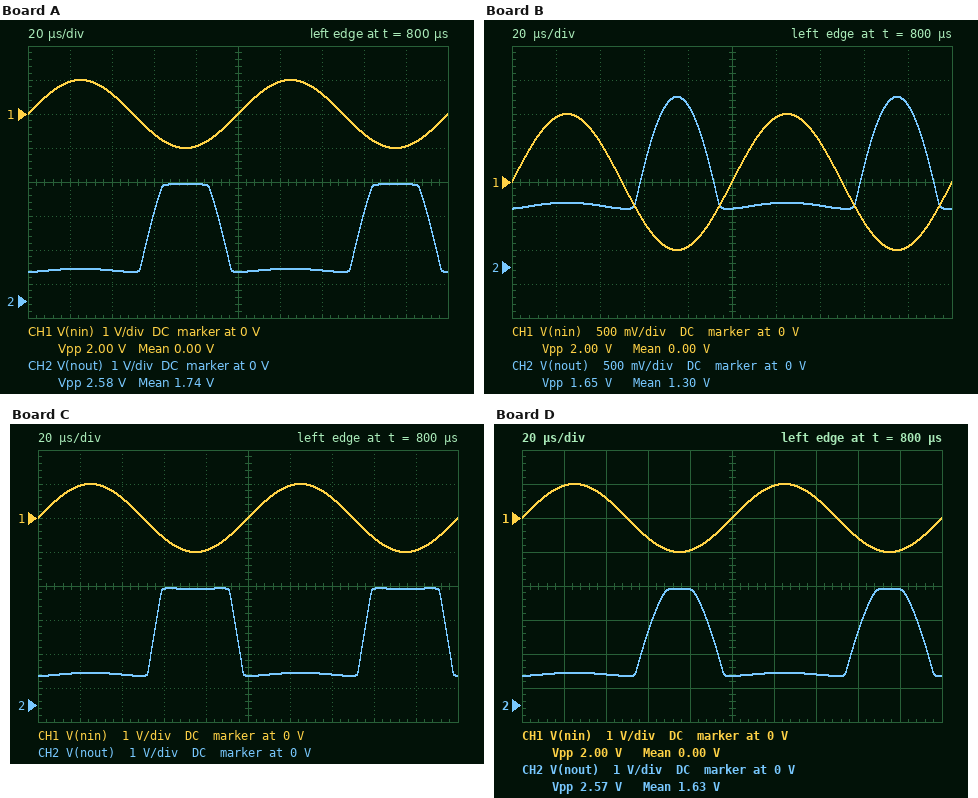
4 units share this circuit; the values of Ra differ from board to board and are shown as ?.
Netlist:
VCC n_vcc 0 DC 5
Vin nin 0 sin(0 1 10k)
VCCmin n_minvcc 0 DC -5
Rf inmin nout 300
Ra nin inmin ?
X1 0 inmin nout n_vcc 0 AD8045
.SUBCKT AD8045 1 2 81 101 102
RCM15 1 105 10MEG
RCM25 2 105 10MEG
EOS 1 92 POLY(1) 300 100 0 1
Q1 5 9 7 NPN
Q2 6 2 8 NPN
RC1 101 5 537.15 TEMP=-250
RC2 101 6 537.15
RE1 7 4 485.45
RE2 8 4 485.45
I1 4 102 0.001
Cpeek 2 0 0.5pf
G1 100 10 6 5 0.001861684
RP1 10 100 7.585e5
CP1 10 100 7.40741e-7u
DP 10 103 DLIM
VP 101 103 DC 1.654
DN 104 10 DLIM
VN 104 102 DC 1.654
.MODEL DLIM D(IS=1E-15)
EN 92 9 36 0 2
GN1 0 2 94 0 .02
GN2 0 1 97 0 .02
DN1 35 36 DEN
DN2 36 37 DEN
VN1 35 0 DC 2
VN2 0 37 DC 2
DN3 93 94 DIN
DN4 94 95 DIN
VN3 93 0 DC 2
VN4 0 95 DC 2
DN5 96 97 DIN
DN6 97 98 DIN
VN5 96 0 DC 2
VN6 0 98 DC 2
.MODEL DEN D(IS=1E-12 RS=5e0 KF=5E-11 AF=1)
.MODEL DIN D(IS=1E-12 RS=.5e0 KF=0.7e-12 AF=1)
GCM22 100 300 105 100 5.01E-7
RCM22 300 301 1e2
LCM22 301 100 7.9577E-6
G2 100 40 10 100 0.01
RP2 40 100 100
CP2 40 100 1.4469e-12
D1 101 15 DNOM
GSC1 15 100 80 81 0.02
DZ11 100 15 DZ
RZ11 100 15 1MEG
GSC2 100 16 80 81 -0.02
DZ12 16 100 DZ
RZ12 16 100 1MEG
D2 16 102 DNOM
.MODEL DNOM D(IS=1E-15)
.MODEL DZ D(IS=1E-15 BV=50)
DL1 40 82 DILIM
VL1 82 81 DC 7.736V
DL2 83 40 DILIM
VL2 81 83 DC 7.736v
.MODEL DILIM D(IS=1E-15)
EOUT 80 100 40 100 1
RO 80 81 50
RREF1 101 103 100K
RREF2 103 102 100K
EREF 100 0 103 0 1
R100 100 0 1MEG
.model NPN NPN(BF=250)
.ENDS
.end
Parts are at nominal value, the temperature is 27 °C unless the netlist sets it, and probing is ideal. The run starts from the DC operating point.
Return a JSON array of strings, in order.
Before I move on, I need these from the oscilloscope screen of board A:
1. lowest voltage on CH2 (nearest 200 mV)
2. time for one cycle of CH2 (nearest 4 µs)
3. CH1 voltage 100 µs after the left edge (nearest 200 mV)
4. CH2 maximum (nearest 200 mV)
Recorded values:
["800 mV", "100 µs", "0 V", "3.4 V"]
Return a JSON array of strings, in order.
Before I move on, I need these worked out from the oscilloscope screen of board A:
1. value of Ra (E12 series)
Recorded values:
["68 Ω"]
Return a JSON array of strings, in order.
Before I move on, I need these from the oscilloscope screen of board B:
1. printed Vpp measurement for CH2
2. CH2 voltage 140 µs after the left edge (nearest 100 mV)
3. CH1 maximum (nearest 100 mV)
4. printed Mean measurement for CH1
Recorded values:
["1.65 V", "900 mV", "1.0 V", "0.00 V"]
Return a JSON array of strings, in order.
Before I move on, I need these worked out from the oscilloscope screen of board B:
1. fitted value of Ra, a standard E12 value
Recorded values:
["120 Ω"]
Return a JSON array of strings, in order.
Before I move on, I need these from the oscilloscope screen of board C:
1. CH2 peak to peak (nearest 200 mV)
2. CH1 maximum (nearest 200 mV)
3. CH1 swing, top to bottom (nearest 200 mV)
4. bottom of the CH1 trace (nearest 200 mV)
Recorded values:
["2.6 V", "1.0 V", "2.0 V", "-1.0 V"]
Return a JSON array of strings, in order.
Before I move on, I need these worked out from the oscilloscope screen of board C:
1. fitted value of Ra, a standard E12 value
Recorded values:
["47 Ω"]
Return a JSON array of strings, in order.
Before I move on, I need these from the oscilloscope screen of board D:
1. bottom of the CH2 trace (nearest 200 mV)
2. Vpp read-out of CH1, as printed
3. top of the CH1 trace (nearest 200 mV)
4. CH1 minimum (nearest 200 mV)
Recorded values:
["800 mV", "2.00 V", "1.0 V", "-1.0 V"]
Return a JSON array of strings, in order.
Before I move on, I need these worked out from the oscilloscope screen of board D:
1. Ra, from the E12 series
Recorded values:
["82 Ω"]
